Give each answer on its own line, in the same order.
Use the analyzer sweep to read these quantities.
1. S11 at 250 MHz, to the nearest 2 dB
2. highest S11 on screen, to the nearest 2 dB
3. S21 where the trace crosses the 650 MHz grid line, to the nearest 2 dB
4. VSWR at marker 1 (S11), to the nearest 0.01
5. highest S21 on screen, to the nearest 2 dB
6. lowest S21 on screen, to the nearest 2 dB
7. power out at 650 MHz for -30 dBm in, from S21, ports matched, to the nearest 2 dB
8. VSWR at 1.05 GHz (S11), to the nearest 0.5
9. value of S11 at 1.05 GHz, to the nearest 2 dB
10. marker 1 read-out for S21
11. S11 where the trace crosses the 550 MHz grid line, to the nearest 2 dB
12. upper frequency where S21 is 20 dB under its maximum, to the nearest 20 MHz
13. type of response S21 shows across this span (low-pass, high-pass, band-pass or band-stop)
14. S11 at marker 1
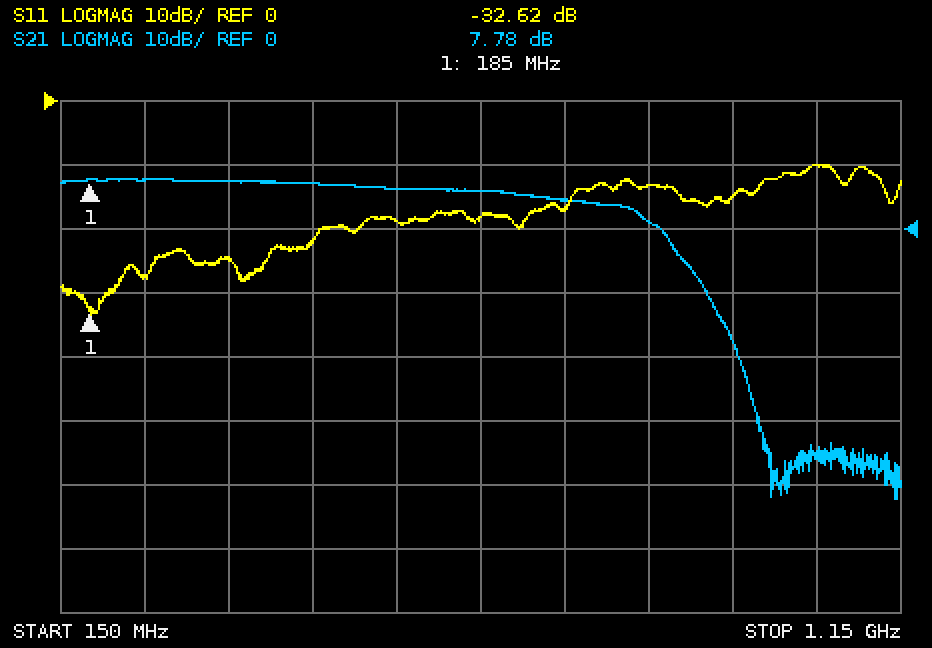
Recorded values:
-28 dB
-10 dB
6 dB
1.05
8 dB
-42 dB
-24 dBm
2.0
-10 dB
7.78 dB
-18 dB
920 MHz
low-pass
-32.62 dB
